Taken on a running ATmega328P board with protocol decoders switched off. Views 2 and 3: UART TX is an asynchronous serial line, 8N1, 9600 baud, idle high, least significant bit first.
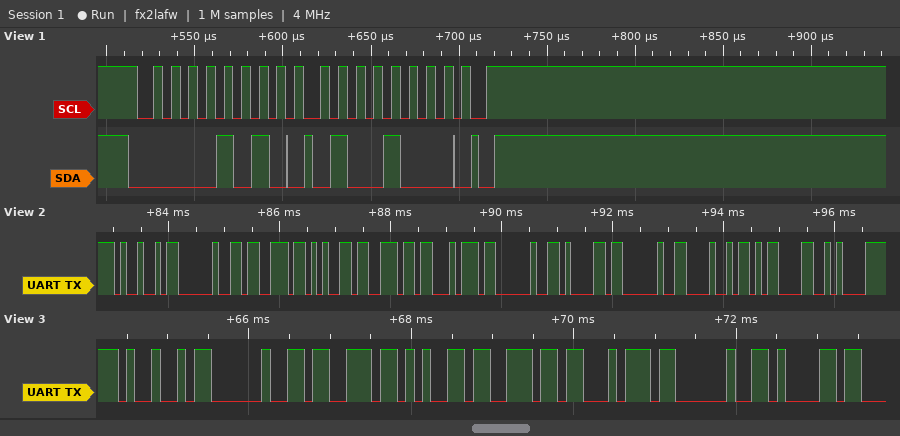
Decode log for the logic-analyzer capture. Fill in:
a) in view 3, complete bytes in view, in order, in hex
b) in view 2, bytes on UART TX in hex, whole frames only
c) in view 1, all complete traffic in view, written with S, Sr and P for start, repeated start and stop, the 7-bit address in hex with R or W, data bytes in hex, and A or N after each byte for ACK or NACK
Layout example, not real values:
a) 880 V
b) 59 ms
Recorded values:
a) 0x49 0x20 0x73 0x65 0x6E 0x74 0x20 0x61
b) 49 20 73 65 6E 74 20 61 20 48 0D 0A
c) S 05W A 48 A P
